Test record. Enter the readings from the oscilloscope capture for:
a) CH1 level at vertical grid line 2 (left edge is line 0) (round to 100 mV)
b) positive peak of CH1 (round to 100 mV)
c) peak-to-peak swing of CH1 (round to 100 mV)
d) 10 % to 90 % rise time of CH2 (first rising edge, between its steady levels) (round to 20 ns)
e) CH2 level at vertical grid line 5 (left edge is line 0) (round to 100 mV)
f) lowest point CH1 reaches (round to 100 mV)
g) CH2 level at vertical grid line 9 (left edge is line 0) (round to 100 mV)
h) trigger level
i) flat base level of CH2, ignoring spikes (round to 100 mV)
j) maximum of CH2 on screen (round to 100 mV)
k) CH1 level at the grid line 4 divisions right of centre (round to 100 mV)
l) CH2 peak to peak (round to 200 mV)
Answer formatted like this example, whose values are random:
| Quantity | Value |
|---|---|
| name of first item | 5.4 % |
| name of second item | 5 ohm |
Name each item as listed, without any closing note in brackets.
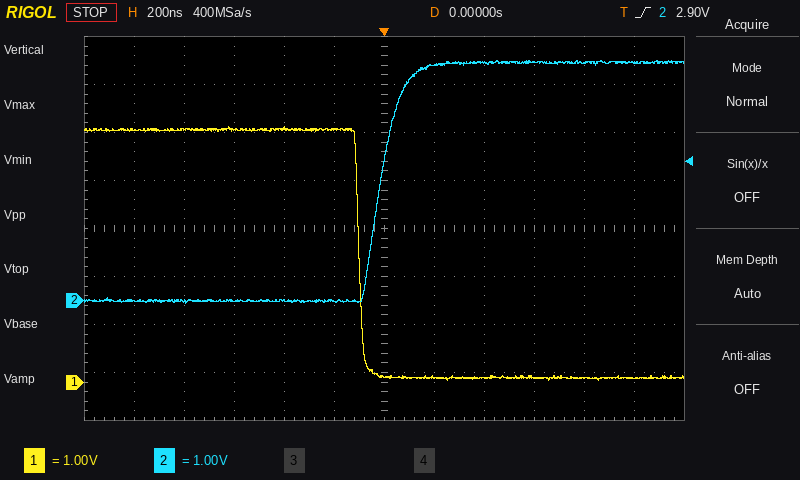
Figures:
| Quantity | Value |
|---|---|
| CH1 level at vertical grid line 2 (left edge is line 0) | 5.3 V |
| positive peak of CH1 | 5.3 V |
| peak-to-peak swing of CH1 | 5.3 V |
| 10 % to 90 % rise time of CH2 (first rising edge, between its steady levels) | 160 ns |
| CH2 level at vertical grid line 5 (left edge is line 0) | 0.0 V |
| lowest point CH1 reaches | 0.0 V |
| CH2 level at vertical grid line 9 (left edge is line 0) | 5.0 V |
| trigger level | 2.90 V |
| flat base level of CH2, ignoring spikes | 0.0 V |
| maximum of CH2 on screen | 5.0 V |
| CH1 level at the grid line 4 divisions right of centre | 100 mV |
| CH2 peak to peak | 5.0 V |
